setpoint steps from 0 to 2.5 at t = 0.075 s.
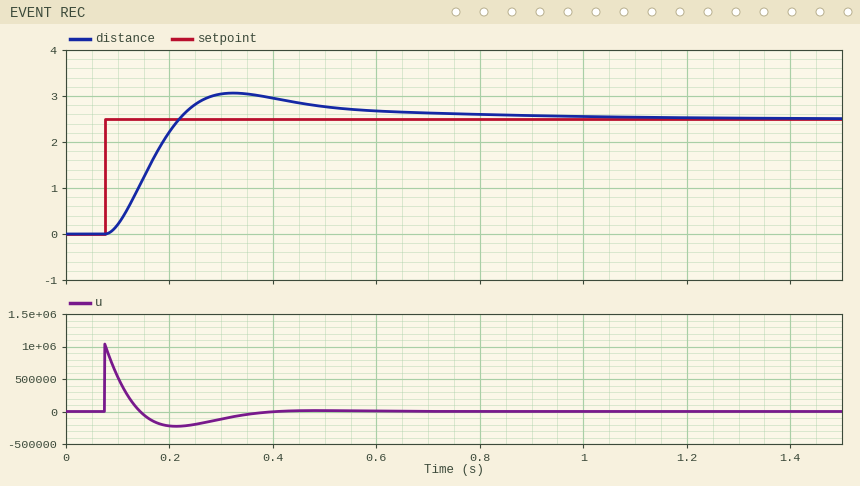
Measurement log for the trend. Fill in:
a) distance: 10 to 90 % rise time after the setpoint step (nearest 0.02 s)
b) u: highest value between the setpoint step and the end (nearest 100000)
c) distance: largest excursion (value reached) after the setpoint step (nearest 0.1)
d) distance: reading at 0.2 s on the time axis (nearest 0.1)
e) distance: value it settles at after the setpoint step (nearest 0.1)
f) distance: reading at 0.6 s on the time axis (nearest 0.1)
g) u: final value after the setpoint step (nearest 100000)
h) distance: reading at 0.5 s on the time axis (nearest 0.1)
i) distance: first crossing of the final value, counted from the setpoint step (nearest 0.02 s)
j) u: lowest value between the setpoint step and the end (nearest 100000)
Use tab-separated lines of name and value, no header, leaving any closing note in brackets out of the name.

distance: 10 to 90 % rise time after the setpoint step	0.10 s
u: highest value between the setpoint step and the end	1000000
distance: largest excursion (value reached) after the setpoint step	3.1
distance: reading at 0.2 s on the time axis	2.2
distance: value it settles at after the setpoint step	2.5
distance: reading at 0.6 s on the time axis	2.7
u: final value after the setpoint step	0
distance: reading at 0.5 s on the time axis	2.8
distance: first crossing of the final value, counted from the setpoint step	0.14 s
u: lowest value between the setpoint step and the end	-200000
